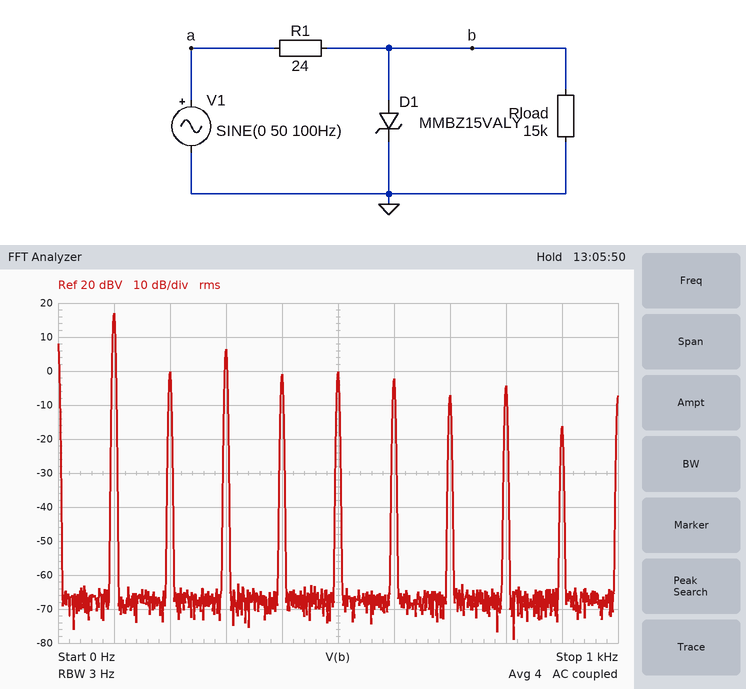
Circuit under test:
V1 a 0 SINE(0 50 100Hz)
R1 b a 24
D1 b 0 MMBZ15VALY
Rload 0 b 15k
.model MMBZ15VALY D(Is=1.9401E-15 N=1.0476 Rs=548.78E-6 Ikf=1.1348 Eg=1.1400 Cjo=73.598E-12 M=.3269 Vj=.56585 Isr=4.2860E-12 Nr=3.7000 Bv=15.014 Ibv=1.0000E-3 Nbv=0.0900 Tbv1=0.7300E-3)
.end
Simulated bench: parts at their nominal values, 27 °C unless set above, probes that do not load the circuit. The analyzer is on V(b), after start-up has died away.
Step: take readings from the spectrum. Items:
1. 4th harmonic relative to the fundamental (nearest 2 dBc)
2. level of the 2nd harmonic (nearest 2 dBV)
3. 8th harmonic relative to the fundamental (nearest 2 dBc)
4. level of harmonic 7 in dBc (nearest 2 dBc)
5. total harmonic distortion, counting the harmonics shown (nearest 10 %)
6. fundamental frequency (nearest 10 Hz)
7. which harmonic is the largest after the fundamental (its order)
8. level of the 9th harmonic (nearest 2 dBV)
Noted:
-18 dBc
0 dBV
-22 dBc
-24 dBc
40 %
100 Hz
3
-16 dBV
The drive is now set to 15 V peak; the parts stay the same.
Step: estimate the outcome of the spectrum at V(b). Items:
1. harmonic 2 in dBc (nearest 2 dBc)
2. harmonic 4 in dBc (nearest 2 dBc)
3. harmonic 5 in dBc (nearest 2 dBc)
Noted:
-8 dBc
-22 dBc
-38 dBc
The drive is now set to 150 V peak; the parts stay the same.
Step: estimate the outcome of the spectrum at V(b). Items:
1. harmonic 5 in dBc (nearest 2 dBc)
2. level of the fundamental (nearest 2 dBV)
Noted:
-14 dBc
18 dBV
